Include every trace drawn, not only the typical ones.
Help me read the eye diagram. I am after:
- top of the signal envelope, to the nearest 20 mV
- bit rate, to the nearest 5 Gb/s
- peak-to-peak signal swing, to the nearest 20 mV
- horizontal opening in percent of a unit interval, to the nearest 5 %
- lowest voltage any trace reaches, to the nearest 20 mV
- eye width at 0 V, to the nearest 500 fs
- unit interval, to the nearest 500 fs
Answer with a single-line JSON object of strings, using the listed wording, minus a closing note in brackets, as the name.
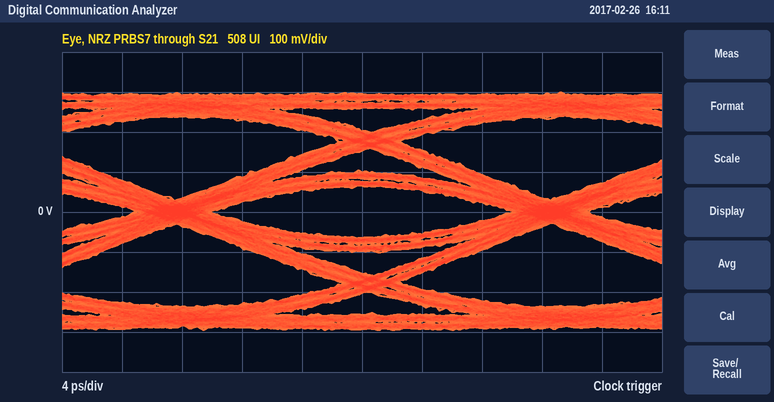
{"top of the signal envelope, to the nearest 20 mV": "300 mV", "bit rate, to the nearest 5 Gb/s": "40 Gb/s", "peak-to-peak signal swing, to the nearest 20 mV": "600 mV", "horizontal opening in percent of a unit interval, to the nearest 5 %": "80 %", "lowest voltage any trace reaches, to the nearest 20 mV": "-300 mV", "eye width at 0 V, to the nearest 500 fs": "20.0 ps", "unit interval, to the nearest 500 fs": "25.0 ps"}
